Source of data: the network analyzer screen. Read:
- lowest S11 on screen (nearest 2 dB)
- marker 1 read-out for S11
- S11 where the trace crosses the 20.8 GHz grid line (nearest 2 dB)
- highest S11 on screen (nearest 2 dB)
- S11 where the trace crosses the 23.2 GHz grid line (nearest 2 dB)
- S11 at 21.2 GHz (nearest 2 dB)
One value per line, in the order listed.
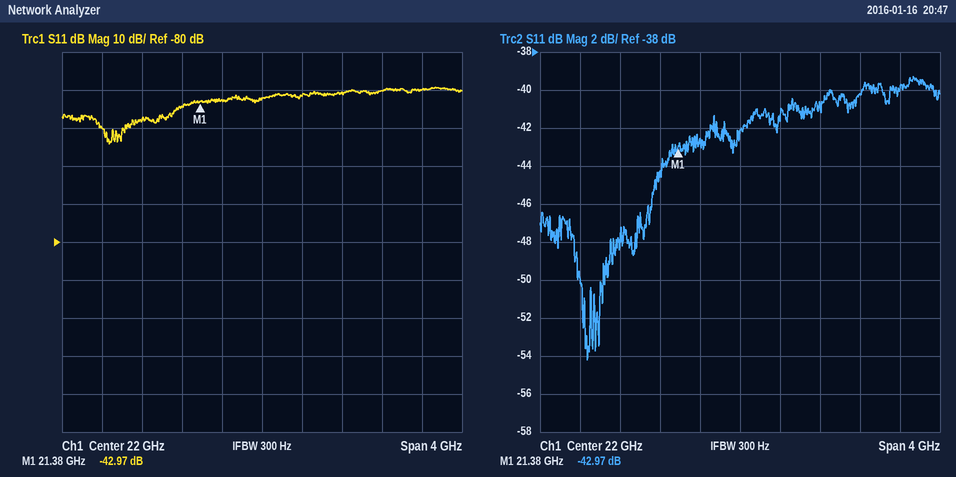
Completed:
-54 dB
-42.97 dB
-48 dB
-40 dB
-40 dB
-44 dB
